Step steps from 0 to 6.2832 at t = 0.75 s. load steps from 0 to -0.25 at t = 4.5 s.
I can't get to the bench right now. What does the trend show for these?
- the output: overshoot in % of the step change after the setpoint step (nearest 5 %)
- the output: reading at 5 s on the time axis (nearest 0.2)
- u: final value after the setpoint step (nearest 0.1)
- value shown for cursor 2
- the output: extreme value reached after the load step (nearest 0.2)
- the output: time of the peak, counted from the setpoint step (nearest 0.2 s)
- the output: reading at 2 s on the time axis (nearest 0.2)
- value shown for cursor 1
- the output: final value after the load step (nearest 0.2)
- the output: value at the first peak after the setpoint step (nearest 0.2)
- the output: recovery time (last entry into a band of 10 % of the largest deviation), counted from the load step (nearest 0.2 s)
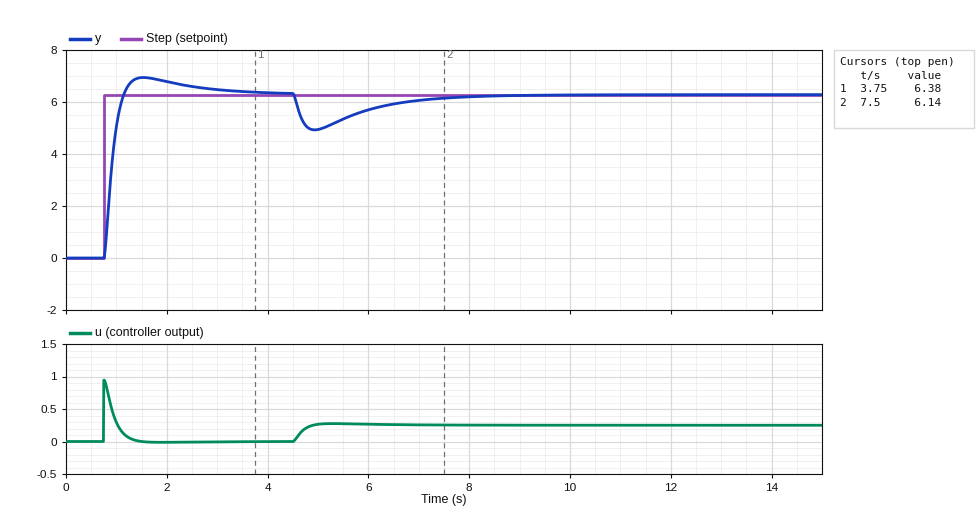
10 %
5.0
0.0
6.14
5.0
0.8 s
6.8
6.38
6.2
7.0
3.0 s
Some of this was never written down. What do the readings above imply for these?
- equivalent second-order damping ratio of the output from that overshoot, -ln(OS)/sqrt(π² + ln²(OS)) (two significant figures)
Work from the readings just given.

0.59
